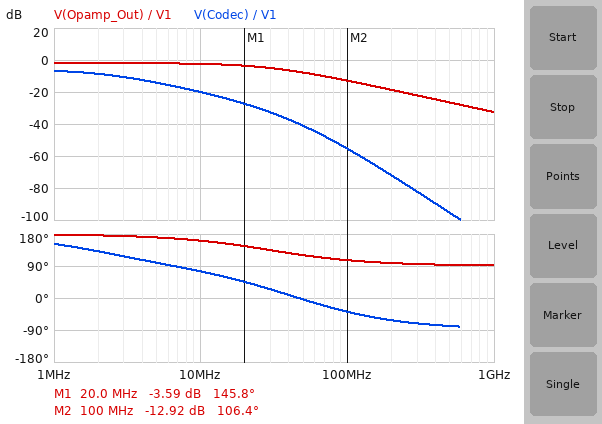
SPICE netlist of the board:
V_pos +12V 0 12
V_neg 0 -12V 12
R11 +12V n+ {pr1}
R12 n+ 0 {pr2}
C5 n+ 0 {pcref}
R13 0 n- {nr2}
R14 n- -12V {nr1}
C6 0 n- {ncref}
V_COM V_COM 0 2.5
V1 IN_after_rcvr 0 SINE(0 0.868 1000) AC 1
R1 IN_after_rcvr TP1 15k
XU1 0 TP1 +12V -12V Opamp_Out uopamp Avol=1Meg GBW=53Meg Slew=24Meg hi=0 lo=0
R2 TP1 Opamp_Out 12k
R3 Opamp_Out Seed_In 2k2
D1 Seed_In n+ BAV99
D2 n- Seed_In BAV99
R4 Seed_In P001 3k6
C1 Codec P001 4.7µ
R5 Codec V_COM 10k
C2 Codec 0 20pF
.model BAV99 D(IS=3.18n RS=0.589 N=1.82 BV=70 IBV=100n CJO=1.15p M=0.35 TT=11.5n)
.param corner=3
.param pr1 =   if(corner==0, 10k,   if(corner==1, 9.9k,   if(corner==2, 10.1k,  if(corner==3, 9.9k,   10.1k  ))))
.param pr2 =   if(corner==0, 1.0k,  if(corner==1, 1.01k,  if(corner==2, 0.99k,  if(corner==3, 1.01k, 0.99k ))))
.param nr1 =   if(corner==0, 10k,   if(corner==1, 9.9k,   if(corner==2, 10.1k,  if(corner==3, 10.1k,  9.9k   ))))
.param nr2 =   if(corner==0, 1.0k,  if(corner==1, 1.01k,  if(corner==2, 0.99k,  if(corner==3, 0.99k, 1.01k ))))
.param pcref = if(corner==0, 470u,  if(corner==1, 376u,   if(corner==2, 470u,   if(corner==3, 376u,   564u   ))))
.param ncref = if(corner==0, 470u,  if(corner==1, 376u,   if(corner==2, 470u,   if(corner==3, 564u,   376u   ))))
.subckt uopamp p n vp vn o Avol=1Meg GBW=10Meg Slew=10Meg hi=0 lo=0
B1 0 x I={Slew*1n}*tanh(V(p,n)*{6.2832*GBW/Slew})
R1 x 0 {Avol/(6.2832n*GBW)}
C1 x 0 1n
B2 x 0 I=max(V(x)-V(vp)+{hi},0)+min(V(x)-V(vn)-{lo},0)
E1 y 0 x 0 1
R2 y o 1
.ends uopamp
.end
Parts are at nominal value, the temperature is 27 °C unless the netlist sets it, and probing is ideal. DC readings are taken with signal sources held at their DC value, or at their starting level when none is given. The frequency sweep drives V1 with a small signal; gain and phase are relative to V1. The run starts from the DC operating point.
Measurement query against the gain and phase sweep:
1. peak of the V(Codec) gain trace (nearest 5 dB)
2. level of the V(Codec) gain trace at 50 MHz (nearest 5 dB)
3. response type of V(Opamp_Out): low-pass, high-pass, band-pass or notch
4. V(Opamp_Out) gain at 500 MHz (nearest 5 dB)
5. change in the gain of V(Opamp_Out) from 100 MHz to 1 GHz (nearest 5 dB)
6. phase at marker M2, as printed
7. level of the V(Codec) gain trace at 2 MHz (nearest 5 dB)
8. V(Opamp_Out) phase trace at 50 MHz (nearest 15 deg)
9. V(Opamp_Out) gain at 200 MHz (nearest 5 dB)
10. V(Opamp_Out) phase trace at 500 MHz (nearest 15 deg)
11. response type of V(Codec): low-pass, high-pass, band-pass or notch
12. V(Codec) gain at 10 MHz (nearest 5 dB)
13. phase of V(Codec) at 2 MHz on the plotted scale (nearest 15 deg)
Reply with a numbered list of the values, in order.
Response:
1. -5 dB
2. -40 dB
3. low-pass
4. -25 dB
5. -20 dB
6. 106.4 deg
7. -10 dB
8. 120 deg
9. -20 dB
10. 90 deg
11. low-pass
12. -20 dB
13. 135 deg
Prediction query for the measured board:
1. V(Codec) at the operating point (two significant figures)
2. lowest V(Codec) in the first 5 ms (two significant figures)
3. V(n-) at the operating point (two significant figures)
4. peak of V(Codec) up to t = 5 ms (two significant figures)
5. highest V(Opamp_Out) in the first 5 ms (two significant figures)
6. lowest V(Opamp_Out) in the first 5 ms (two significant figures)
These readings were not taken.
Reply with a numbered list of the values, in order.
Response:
1. 2.5 V
2. 2.1 V
3. -1.1 V
4. 2.9 V
5. 690 mV
6. -690 mV
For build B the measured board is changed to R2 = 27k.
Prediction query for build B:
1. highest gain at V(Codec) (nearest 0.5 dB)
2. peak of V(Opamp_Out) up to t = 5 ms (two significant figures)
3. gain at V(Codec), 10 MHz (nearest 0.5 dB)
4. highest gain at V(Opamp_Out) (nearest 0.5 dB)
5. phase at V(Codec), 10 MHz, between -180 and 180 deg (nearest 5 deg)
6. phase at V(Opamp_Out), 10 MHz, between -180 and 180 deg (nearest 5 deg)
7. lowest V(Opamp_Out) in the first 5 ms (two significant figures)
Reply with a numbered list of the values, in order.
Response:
1. 1.0 dB
2. 1.6 V
3. -13.5 dB
4. 5.0 dB
5. 65 deg
6. 150 deg
7. -1.6 V
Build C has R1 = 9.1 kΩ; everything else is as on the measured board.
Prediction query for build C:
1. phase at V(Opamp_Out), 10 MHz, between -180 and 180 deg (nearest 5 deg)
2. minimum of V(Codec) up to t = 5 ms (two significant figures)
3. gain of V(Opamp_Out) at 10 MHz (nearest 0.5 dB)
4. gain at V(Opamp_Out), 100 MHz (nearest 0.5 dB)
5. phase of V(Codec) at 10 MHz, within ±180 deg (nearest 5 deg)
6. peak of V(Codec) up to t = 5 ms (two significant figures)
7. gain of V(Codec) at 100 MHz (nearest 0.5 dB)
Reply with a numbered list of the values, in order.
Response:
1. 155 deg
2. 1.8 V
3. 1.5 dB
4. -10.5 dB
5. 70 deg
6. 3.2 V
7. -53.0 dB
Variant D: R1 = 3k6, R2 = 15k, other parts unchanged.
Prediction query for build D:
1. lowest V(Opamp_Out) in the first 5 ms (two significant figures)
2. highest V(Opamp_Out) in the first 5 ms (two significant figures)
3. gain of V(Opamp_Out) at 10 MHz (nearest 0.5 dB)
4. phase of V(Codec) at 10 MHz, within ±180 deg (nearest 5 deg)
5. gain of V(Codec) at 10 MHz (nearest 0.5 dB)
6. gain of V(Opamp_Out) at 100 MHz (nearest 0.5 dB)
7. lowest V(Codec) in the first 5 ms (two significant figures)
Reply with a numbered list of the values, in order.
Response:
1. -3.6 V
2. 3.6 V
3. 9.5 dB
4. 50 deg
5. -8.0 dB
6. -7.5 dB
7. 1.3 V
